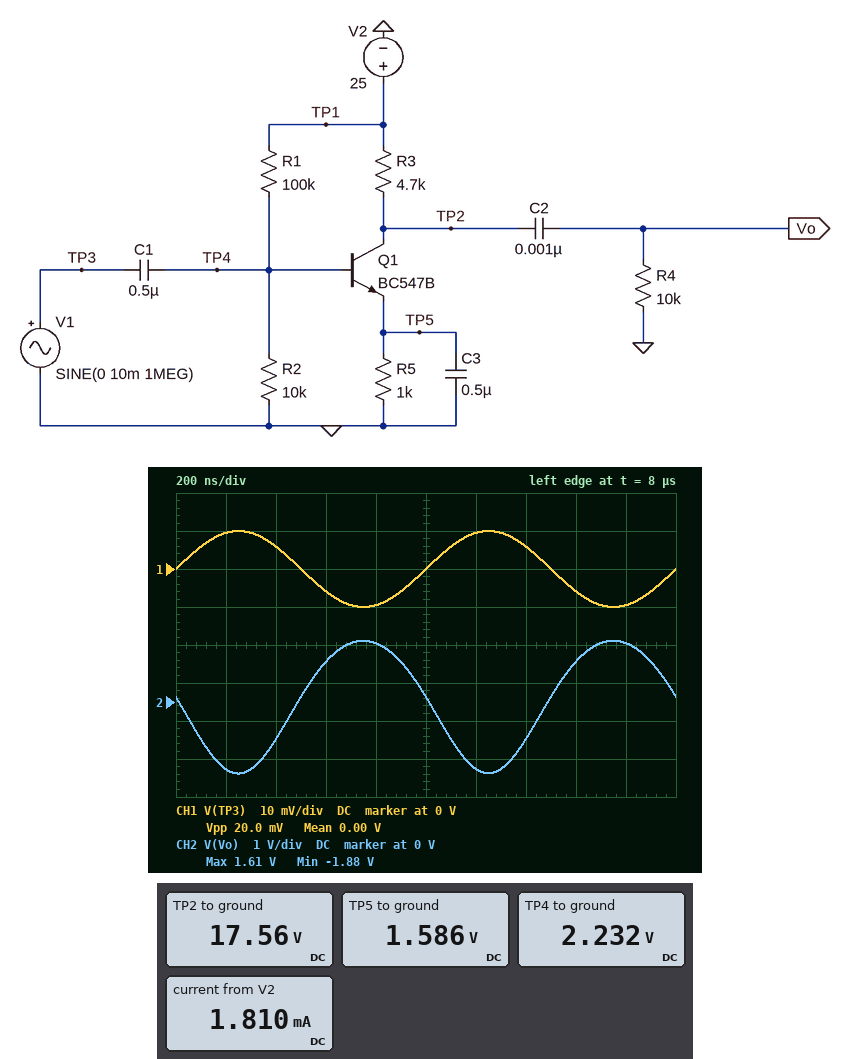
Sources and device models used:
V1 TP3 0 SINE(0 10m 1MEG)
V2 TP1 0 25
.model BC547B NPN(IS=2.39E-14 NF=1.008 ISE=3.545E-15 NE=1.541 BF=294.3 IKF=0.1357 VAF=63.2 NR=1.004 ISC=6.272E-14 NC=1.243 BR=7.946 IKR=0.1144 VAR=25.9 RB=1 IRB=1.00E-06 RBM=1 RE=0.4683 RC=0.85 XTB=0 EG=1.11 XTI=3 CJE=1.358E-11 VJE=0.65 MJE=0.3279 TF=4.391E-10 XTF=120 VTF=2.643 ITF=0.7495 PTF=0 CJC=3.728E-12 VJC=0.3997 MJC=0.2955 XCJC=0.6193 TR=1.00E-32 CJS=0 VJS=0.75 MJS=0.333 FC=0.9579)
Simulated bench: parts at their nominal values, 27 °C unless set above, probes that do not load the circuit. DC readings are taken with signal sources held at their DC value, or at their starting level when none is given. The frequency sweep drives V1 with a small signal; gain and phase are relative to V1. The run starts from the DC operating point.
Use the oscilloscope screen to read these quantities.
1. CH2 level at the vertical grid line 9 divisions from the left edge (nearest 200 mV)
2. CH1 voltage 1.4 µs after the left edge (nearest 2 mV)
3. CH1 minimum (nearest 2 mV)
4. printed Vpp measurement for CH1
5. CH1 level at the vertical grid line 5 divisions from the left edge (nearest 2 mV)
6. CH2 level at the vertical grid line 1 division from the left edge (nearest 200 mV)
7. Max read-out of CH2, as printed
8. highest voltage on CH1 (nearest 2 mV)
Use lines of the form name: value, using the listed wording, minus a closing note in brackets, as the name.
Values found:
CH2 level at the vertical grid line 9 divisions from the left edge: 1.6 V
CH1 voltage 1.4 µs after the left edge: 6 mV
CH1 minimum: -10 mV
printed Vpp measurement for CH1: 20.0 mV
CH1 level at the vertical grid line 5 divisions from the left edge: 0 V
CH2 level at the vertical grid line 1 division from the left edge: -1.8 V
Max read-out of CH2, as printed: 1.61 V
highest voltage on CH1: 10 mV
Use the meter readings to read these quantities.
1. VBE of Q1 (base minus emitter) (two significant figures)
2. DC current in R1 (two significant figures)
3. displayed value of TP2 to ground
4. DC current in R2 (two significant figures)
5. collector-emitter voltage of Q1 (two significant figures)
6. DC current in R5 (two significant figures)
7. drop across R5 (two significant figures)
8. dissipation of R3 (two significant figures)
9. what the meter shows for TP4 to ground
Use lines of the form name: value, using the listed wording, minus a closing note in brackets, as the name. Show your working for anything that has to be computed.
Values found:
VBE of Q1 (base minus emitter): 2.232 V - 1.586 V = 650 mV
DC current in R1: (25 V - 2.232 V) / 100 kΩ = 230 µA
displayed value of TP2 to ground: 17.56 V
DC current in R2: (2.232 V) / 10 kΩ = 220 µA
collector-emitter voltage of Q1: 17.56 V - 1.586 V = 16 V
DC current in R5: (1.586 V) / 1 kΩ = 1.6 mA
drop across R5: 1.586 V = 1.6 V
dissipation of R3: (25 V - 17.56 V)^2 / 4.7 kΩ = 12 mW
what the meter shows for TP4 to ground: 2.232 V
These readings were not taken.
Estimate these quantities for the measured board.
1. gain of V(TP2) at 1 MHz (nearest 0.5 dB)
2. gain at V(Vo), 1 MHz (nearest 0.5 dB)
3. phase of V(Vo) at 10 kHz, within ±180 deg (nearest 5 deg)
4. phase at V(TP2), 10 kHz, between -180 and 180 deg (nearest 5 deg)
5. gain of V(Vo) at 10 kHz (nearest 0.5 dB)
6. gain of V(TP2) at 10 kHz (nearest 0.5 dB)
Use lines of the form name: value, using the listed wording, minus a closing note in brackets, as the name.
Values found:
gain of V(TP2) at 1 MHz: 45.0 dB
gain at V(Vo), 1 MHz: 45.0 dB
phase of V(Vo) at 10 kHz, within ±180 deg: -75 deg
phase at V(TP2), 10 kHz, between -180 and 180 deg: -130 deg
gain of V(Vo) at 10 kHz: 35.0 dB
gain of V(TP2) at 10 kHz: 40.5 dB
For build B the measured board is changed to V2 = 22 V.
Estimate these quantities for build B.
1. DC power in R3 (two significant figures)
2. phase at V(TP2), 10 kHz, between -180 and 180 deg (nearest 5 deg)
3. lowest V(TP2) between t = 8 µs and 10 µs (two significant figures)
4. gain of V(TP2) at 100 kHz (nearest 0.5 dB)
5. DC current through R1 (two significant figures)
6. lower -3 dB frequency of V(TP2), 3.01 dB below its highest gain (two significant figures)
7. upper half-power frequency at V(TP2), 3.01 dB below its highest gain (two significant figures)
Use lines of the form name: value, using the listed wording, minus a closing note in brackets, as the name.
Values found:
DC power in R3: 8.2 mW
phase at V(TP2), 10 kHz, between -180 and 180 deg: -135 deg
lowest V(TP2) between t = 8 µs and 10 µs: 14 V
gain of V(TP2) at 100 kHz: 43.5 dB
DC current through R1: 200 µA
lower -3 dB frequency of V(TP2), 3.01 dB below its highest gain: 10 kHz
upper half-power frequency at V(TP2), 3.01 dB below its highest gain: 39 MHz
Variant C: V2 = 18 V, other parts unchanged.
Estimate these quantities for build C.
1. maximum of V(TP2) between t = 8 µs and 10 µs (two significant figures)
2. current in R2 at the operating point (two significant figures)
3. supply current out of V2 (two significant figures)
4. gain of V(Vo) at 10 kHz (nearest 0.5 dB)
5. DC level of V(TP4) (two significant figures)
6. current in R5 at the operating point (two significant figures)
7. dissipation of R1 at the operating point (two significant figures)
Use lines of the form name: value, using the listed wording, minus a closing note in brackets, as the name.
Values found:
maximum of V(TP2) between t = 8 µs and 10 µs: 14 V
current in R2 at the operating point: 160 µA
supply current out of V2: 1.1 mA
gain of V(Vo) at 10 kHz: 34.0 dB
DC level of V(TP4): 1.6 V
current in R5 at the operating point: 980 µA
dissipation of R1 at the operating point: 2.7 mW
